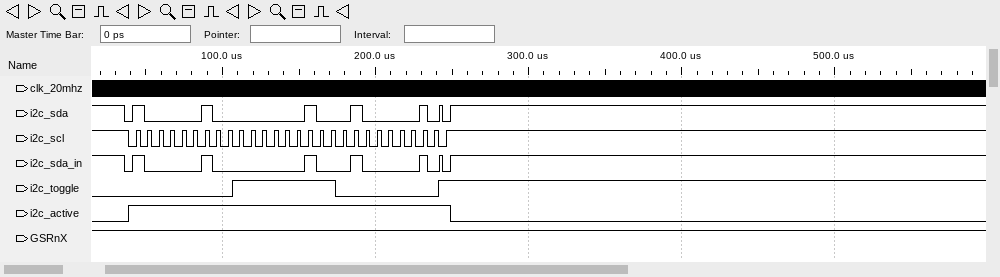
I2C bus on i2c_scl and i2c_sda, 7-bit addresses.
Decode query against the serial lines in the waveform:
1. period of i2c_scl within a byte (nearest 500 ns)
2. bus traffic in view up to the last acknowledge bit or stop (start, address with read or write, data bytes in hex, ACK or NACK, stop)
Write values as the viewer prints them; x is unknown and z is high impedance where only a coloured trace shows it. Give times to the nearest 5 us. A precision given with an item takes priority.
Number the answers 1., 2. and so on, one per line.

1. 7500 ns
2. start, address 41 write ACK, 02 ACK, 41 ACK, stop
